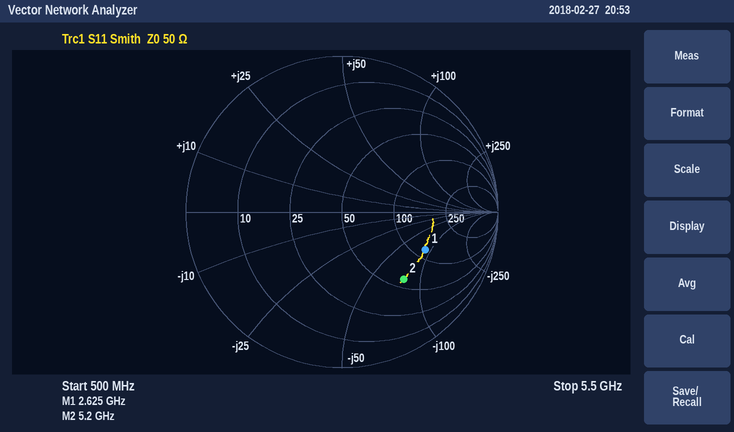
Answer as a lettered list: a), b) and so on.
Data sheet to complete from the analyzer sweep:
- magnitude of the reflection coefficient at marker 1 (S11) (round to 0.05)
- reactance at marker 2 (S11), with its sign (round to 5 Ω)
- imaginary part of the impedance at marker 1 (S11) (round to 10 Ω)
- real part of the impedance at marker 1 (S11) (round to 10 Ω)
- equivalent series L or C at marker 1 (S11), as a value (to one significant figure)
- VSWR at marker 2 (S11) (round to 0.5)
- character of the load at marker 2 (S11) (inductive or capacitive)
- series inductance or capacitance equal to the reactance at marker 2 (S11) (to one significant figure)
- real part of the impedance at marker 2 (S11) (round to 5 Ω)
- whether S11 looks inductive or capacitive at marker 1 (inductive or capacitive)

a) 0.60
b) -80 Ω
c) -90 Ω
d) 120 Ω
e) 700 fF
f) 4.0
g) capacitive
h) 400 fF
i) 60 Ω
j) capacitive
